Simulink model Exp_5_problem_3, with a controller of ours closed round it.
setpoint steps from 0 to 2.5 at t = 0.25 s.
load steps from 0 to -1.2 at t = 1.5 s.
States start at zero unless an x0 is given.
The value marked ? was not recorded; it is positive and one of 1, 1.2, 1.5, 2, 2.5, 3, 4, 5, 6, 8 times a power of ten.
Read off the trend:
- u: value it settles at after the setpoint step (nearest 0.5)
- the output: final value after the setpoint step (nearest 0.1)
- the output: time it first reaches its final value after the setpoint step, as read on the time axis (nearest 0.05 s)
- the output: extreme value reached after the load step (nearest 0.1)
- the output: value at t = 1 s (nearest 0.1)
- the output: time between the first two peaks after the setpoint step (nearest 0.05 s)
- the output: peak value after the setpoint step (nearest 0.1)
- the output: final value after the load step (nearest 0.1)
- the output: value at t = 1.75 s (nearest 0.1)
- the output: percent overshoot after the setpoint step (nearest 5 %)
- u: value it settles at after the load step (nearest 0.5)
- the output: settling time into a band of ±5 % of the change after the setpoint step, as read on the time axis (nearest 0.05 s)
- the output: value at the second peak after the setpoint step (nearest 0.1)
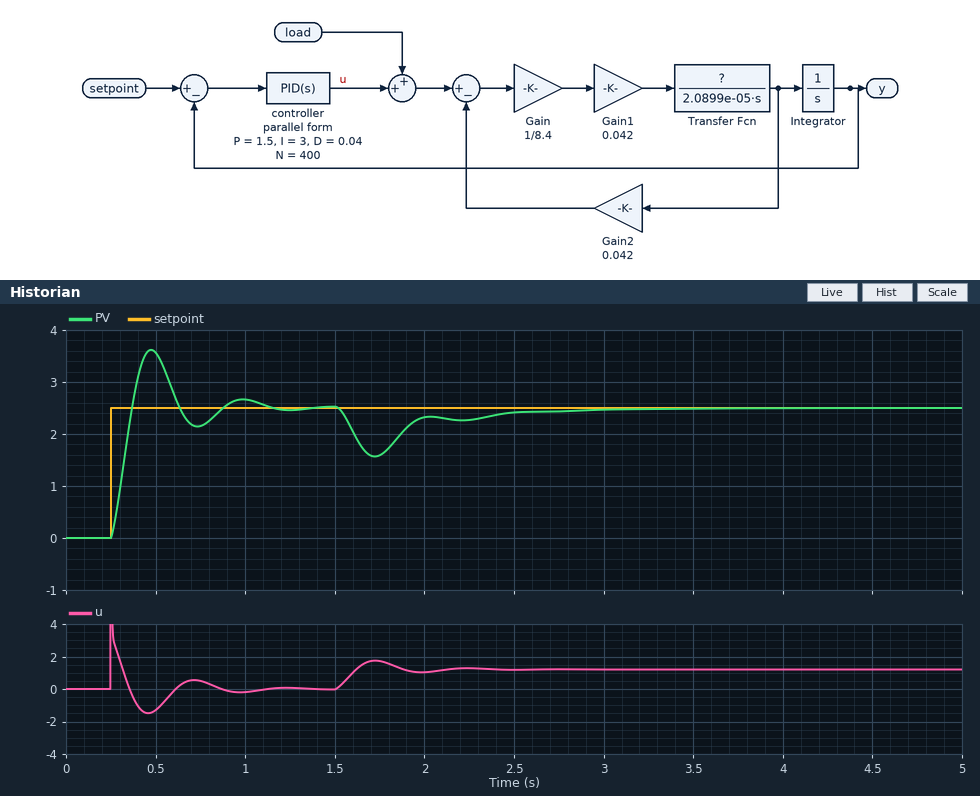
0.0
2.5
0.35 s
1.6
2.7
0.50 s
3.6
2.5
1.6
45 %
1.0
1.05 s
2.7
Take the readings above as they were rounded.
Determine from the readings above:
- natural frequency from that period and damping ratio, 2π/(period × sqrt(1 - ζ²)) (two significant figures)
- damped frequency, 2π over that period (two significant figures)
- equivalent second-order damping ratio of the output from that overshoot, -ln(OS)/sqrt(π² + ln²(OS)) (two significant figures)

13 rad/s
13 rad/s
0.25
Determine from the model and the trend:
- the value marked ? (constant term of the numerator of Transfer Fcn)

0.5
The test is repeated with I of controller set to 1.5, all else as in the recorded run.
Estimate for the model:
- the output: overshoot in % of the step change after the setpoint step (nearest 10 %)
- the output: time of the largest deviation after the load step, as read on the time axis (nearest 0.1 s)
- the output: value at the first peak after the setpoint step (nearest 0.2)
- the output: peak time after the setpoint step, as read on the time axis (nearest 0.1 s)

40 %
1.7 s
3.4
0.5 s
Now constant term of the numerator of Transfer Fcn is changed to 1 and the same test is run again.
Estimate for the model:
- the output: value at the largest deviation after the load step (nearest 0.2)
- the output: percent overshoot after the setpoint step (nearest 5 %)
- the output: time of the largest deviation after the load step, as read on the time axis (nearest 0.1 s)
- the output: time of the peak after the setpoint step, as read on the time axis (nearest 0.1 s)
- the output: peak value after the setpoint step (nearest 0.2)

1.6
25 %
1.7 s
0.4 s
3.2
